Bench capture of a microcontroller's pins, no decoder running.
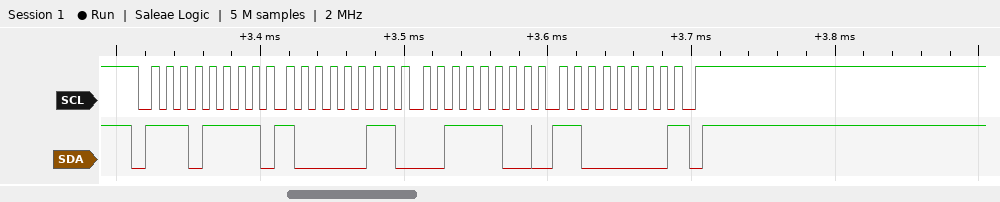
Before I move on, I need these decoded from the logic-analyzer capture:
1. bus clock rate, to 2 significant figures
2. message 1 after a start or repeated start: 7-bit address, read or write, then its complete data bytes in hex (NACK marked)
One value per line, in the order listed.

100 kHz
0x77 read: 83 3C C0 NACK
